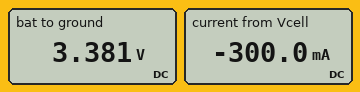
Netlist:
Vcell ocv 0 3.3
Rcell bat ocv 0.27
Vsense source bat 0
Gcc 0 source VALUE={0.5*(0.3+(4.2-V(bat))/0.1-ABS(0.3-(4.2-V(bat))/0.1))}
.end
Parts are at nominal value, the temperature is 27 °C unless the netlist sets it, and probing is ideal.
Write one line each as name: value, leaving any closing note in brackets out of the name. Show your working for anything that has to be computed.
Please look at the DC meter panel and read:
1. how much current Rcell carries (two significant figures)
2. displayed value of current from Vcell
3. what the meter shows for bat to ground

how much current Rcell carries: (3.381 V - 3.3 V) / 270 mΩ = 300 mA
displayed value of current from Vcell: -300.0 mA
what the meter shows for bat to ground: 3.381 V
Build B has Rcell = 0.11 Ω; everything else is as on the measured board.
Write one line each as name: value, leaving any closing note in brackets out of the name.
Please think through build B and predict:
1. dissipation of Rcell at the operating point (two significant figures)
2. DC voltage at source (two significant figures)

dissipation of Rcell at the operating point: 9.9 mW
DC voltage at source: 3.3 V
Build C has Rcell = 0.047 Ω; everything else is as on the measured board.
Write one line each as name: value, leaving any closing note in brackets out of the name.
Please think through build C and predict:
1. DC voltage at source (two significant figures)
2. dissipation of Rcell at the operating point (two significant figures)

DC voltage at source: 3.3 V
dissipation of Rcell at the operating point: 4.2 mW
